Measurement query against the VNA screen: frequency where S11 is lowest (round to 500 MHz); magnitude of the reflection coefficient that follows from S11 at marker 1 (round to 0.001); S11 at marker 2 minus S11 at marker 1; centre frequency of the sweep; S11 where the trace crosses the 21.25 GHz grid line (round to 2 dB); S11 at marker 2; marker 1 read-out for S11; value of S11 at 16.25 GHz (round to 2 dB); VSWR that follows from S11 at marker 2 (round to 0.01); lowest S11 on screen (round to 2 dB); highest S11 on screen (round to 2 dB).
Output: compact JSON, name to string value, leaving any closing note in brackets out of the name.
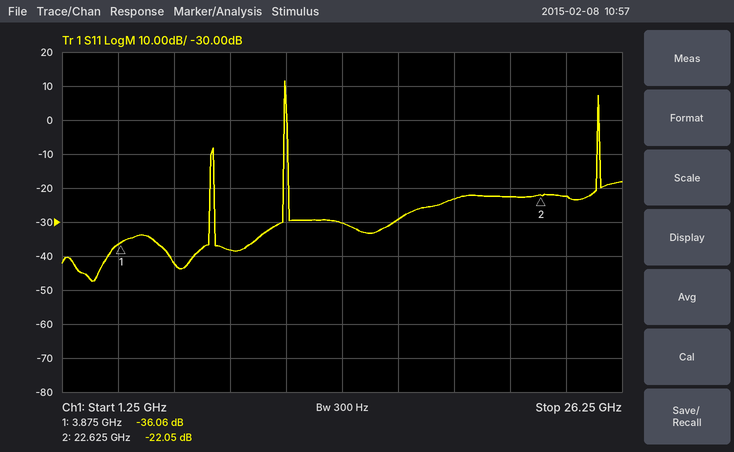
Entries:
{"frequency where S11 is lowest": "2.5 GHz", "magnitude of the reflection coefficient that follows from S11 at marker 1": "0.016", "S11 at marker 2 minus S11 at marker 1": "14.01 dB", "centre frequency of the sweep": "13.75 GHz", "S11 where the trace crosses the 21.25 GHz grid line": "-22 dB", "S11 at marker 2": "-22.05 dB", "marker 1 read-out for S11": "-36.06 dB", "value of S11 at 16.25 GHz": "-30 dB", "VSWR that follows from S11 at marker 2": "1.17", "lowest S11 on screen": "-48 dB", "highest S11 on screen": "12 dB"}
